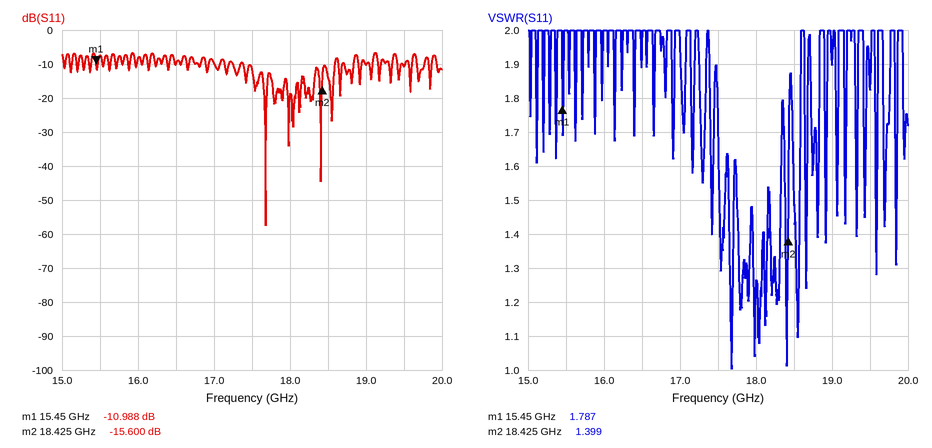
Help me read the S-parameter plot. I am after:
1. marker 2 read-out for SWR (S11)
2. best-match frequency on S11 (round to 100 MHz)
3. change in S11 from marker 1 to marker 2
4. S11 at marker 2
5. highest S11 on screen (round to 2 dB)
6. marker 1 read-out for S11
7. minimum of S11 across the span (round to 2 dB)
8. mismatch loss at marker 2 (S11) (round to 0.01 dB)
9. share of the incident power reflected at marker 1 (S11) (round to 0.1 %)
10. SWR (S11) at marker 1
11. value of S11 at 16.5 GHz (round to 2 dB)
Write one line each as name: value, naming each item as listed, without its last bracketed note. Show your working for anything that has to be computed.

marker 2 read-out for SWR: 1.399
best-match frequency on S11: 17.7 GHz
change in S11 from marker 1 to marker 2: -15.6 − (-10.988) = -4.612 dB
S11 at marker 2: -15.600 dB
highest S11 on screen: -6 dB
marker 1 read-out for S11: -10.988 dB
minimum of S11 across the span: -58 dB
mismatch loss at marker 2 (S11): −10 log10(1 − 10^(-15.6/10)) ≈ 0.12 dB
share of the incident power reflected at marker 1 (S11): 10^(-10.988/10) ≈ 8.0 %
SWR (S11) at marker 1: 1.787
value of S11 at 16.5 GHz: -10 dB
